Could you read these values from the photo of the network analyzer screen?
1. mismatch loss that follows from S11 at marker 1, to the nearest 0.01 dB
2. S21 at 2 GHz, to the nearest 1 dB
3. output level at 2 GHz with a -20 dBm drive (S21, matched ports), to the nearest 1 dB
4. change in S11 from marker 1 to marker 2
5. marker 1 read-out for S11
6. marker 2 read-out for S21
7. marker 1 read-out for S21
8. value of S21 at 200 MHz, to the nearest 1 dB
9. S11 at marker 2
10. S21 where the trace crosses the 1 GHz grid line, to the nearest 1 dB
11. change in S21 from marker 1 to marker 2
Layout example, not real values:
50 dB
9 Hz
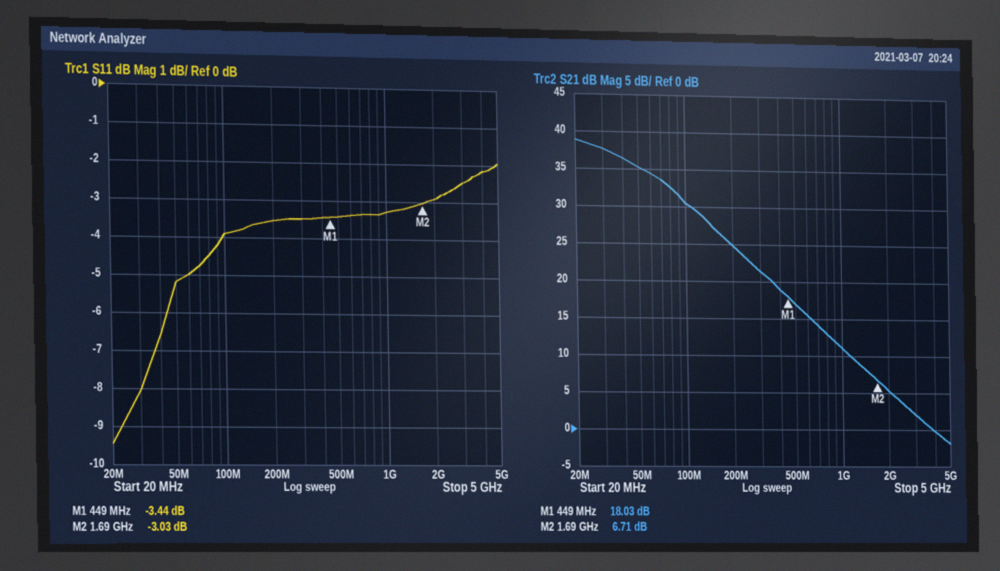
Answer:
2.62 dB
5 dB
-15 dBm
0.41 dB
-3.44 dB
6.71 dB
18.03 dB
25 dB
-3.03 dB
11 dB
-11.32 dB
